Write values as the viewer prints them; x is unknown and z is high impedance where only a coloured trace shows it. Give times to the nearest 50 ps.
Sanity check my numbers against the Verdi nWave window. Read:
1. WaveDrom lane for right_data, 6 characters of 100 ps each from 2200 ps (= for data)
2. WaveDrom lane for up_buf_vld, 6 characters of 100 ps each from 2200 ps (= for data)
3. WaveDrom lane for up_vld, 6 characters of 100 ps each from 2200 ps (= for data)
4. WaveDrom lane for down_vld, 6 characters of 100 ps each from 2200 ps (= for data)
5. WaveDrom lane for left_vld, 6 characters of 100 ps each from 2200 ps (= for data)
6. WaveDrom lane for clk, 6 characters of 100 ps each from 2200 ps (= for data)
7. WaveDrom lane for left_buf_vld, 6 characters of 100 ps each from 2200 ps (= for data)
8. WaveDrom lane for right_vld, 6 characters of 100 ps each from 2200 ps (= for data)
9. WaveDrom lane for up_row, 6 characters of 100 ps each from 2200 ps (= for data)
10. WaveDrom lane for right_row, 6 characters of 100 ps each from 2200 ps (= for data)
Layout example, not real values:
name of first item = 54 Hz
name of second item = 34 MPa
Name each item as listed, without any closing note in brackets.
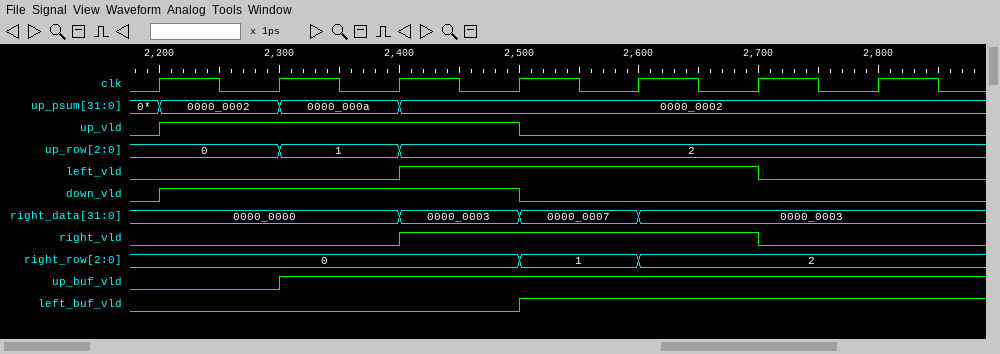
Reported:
WaveDrom lane for right_data, 6 characters of 100 ps each from 2200 ps = {name: 'right_data', wave: '=.===.', data: '0000_0000 0000_0003 0000_0007 0000_0003'}
WaveDrom lane for up_buf_vld, 6 characters of 100 ps each from 2200 ps = {name: 'up_buf_vld', wave: '01....'}
WaveDrom lane for up_vld, 6 characters of 100 ps each from 2200 ps = {name: 'up_vld', wave: '1..0..'}
WaveDrom lane for down_vld, 6 characters of 100 ps each from 2200 ps = {name: 'down_vld', wave: '1..0..'}
WaveDrom lane for left_vld, 6 characters of 100 ps each from 2200 ps = {name: 'left_vld', wave: '0.1..0'}
WaveDrom lane for clk, 6 characters of 100 ps each from 2200 ps = {name: 'clk', wave: 'p.....'}
WaveDrom lane for left_buf_vld, 6 characters of 100 ps each from 2200 ps = {name: 'left_buf_vld', wave: '0..1..'}
WaveDrom lane for right_vld, 6 characters of 100 ps each from 2200 ps = {name: 'right_vld', wave: '0.1..0'}
WaveDrom lane for up_row, 6 characters of 100 ps each from 2200 ps = {name: 'up_row', wave: '===...', data: '0 1 2'}
WaveDrom lane for right_row, 6 characters of 100 ps each from 2200 ps = {name: 'right_row', wave: '=..==.', data: '0 1 2'}
